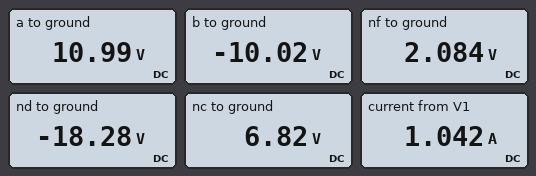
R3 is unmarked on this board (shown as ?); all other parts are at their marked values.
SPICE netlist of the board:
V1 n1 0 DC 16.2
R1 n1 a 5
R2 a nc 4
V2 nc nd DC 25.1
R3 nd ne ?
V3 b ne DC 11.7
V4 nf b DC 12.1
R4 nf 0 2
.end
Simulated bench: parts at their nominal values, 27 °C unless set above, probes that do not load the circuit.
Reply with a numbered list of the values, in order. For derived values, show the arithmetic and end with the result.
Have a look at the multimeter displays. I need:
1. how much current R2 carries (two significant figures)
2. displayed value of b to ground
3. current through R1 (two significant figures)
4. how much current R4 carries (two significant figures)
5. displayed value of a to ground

1. (10.99 V - 6.82 V) / 4 Ω = 1.0 A
2. -10.02 V
3. (16.2 V - 10.99 V) / 5 Ω = 1.0 A
4. (2.084 V) / 2 Ω = 1.0 A
5. 10.99 V
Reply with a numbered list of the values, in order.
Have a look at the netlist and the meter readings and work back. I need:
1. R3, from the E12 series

1. 3.3 Ω
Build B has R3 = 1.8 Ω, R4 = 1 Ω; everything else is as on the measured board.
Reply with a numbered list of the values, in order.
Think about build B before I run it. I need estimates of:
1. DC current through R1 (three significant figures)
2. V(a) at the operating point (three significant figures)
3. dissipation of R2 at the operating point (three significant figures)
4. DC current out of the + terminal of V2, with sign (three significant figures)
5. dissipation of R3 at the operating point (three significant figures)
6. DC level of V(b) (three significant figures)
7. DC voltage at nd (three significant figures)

1. 1.26 A
2. 9.89 V
3. 6.38 W
4. -1.26 A
5. 2.87 W
6. -10.8 V
7. -20.3 V
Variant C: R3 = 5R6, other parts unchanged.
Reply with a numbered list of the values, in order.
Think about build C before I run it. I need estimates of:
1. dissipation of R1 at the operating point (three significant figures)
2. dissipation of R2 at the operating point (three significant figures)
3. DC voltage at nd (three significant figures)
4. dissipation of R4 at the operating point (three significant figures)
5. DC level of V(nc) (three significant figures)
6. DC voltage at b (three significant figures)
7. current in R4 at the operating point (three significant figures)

1. 4.03 W
2. 3.22 W
3. -17.0 V
4. 1.61 W
5. 8.12 V
6. -10.3 V
7. 898 mA
